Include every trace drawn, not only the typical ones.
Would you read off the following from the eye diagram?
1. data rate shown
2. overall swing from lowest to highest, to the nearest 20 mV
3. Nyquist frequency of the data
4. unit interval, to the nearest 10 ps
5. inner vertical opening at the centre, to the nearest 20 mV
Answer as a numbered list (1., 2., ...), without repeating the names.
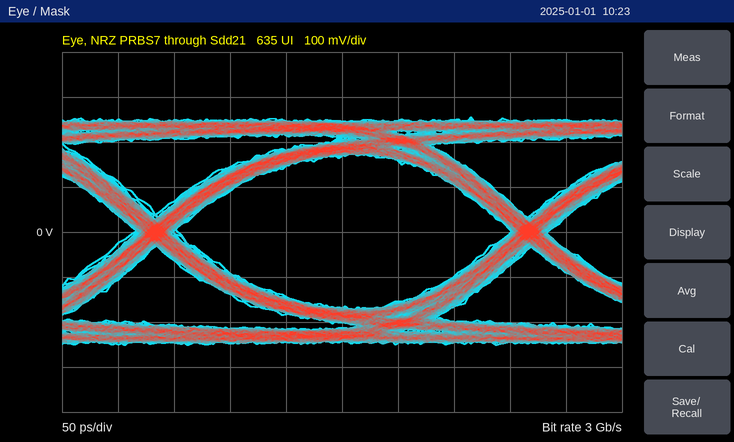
1. 3 Gb/s
2. 500 mV
3. 1.5 GHz
4. 330 ps
5. 340 mV
